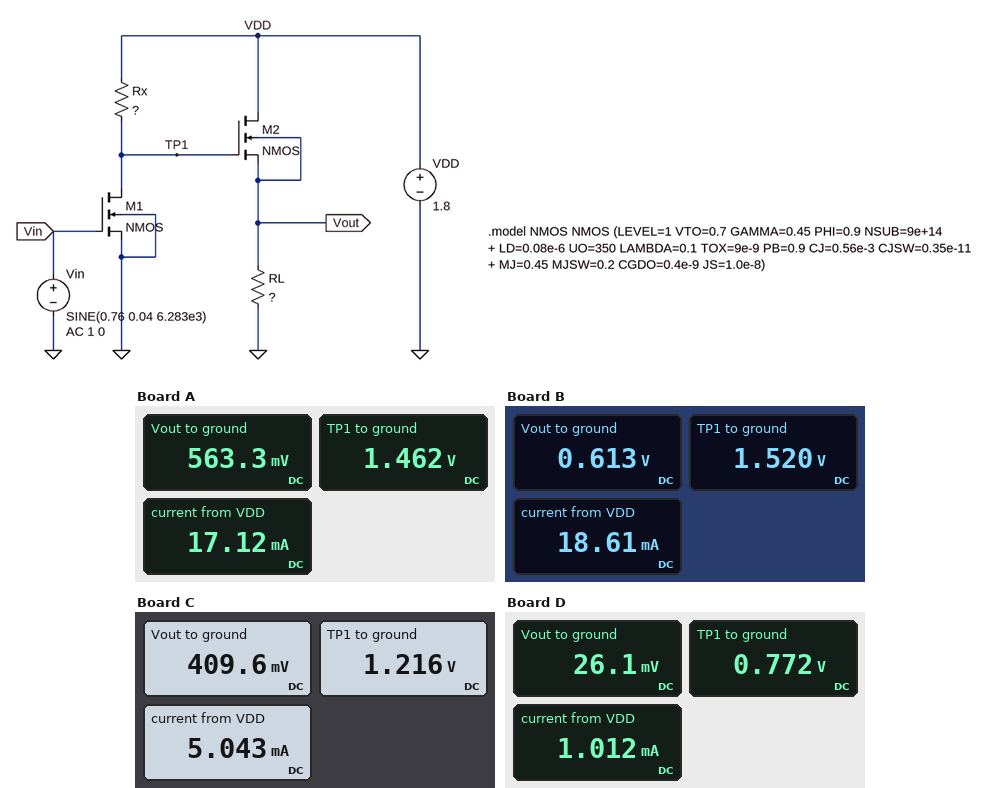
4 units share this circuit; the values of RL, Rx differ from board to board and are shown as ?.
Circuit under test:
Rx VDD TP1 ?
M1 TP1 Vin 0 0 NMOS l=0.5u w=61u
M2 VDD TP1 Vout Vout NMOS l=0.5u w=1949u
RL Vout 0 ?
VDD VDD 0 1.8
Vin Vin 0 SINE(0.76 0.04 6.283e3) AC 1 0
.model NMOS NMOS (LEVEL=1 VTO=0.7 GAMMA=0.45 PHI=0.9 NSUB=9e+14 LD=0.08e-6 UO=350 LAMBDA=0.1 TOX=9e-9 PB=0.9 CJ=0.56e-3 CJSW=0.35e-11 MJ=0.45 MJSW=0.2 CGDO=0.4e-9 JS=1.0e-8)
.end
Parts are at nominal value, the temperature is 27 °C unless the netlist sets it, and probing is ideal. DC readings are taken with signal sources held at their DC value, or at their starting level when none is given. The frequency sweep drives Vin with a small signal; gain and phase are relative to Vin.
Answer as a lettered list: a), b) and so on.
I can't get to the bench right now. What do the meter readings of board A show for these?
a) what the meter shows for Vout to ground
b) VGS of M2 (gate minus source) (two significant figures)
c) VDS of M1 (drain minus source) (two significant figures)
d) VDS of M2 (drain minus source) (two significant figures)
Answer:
a) 563.3 mV
b) 900 mV
c) 1.5 V
d) 1.2 V
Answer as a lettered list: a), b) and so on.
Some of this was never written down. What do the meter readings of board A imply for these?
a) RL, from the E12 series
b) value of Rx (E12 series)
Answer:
a) 33 Ω
b) 6.8 kΩ
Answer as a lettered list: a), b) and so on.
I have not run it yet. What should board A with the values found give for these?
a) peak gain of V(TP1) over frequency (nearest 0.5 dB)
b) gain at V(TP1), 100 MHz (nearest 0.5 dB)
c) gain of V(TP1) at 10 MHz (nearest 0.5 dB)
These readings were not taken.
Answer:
a) 21.0 dB
b) 7.5 dB
c) 20.0 dB
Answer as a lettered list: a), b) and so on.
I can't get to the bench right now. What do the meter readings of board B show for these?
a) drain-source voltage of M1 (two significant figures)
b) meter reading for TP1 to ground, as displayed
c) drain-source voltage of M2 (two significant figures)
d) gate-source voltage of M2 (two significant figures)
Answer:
a) 1.5 V
b) 1.520 V
c) 1.2 V
d) 910 mV
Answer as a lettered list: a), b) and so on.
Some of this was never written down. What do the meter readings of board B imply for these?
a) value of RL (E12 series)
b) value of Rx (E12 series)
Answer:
a) 33 Ω
b) 5.6 kΩ
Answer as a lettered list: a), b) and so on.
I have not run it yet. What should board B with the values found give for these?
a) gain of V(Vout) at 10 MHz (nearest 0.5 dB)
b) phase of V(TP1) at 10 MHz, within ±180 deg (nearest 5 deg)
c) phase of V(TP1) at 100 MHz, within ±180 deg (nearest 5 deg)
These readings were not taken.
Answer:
a) 17.0 dB
b) 160 deg
c) 105 deg
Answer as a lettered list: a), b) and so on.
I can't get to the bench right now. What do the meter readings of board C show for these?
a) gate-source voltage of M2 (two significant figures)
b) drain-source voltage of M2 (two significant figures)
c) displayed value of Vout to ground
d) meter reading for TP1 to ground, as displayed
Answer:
a) 810 mV
b) 1.4 V
c) 409.6 mV
d) 1.216 V
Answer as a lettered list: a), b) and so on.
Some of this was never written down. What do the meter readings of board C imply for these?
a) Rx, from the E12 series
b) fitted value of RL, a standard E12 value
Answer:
a) 12 kΩ
b) 82 Ω
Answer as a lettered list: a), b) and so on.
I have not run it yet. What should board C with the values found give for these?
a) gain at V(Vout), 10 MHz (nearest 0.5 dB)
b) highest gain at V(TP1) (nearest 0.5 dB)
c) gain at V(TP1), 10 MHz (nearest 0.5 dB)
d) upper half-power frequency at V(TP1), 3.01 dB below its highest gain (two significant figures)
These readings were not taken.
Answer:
a) 22.5 dB
b) 25.5 dB
c) 23.5 dB
d) 14 MHz
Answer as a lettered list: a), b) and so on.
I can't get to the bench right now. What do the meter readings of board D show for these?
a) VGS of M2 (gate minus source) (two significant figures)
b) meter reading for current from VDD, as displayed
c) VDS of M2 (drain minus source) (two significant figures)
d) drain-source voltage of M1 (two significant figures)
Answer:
a) 750 mV
b) 1.012 mA
c) 1.8 V
d) 770 mV
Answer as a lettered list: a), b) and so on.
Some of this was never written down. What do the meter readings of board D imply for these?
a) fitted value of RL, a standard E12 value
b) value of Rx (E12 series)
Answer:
a) 27 Ω
b) 22 kΩ
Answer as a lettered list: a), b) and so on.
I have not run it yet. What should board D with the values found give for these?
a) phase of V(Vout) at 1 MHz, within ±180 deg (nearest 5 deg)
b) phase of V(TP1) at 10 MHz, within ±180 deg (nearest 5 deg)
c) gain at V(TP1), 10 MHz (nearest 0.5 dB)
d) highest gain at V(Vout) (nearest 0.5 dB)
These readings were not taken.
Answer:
a) 170 deg
b) 115 deg
c) 23.0 dB
d) 24.5 dB
